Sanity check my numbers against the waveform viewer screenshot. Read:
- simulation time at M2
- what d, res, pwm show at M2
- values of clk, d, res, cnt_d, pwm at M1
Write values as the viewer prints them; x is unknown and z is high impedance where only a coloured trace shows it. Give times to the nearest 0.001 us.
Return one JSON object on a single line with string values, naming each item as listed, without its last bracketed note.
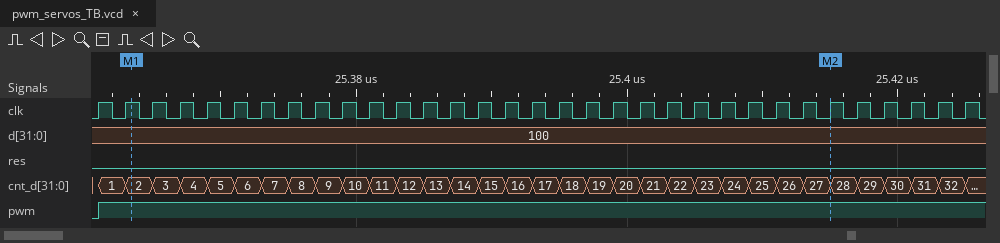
{"simulation time at M2": "25.415 us", "what d, res, pwm show at M2": "d=100, res=0, pwm=1", "values of clk, d, res, cnt_d, pwm at M1": "clk=1, d=100, res=0, cnt_d=2, pwm=1"}
